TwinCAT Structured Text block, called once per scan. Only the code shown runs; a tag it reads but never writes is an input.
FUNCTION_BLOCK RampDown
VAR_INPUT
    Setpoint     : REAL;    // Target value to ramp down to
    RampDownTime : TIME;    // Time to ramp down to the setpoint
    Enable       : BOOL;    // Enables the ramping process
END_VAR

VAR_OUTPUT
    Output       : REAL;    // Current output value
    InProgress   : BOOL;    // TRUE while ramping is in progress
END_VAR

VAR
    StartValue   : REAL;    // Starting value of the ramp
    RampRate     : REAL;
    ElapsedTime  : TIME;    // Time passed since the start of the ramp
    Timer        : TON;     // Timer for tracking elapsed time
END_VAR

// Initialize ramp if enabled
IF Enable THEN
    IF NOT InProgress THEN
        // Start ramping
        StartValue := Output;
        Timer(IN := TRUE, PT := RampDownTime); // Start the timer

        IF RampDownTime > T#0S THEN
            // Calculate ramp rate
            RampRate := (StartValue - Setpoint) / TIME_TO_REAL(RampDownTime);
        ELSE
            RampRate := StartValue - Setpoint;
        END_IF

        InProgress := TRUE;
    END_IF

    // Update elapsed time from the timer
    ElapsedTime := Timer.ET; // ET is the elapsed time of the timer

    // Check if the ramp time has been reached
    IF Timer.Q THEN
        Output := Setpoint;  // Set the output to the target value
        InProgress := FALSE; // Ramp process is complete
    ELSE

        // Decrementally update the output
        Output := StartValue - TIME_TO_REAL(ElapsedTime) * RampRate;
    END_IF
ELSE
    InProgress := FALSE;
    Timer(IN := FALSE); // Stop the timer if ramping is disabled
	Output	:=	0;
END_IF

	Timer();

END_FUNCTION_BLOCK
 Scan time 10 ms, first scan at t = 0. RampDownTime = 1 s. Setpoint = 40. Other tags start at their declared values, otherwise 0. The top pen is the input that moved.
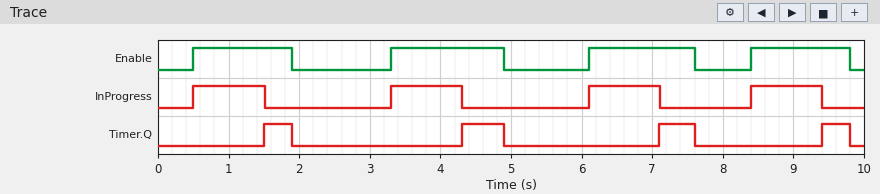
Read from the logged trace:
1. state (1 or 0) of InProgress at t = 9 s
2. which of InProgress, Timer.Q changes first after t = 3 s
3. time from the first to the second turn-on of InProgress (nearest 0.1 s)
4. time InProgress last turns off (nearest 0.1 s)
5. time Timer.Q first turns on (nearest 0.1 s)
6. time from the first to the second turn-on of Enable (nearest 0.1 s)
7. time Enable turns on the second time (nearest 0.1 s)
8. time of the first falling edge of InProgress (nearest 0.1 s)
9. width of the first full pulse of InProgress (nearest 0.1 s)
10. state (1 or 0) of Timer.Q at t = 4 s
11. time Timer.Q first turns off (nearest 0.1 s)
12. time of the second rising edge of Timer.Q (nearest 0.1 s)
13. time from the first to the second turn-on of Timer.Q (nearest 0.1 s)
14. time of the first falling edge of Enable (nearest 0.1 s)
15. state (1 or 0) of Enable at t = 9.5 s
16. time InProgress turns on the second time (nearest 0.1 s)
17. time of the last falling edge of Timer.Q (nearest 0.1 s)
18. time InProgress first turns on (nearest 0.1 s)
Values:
1
InProgress
2.8 s
9.4 s
1.5 s
2.8 s
3.3 s
1.5 s
1.0 s
0
1.9 s
4.3 s
2.8 s
1.9 s
1
3.3 s
9.8 s
0.5 s
